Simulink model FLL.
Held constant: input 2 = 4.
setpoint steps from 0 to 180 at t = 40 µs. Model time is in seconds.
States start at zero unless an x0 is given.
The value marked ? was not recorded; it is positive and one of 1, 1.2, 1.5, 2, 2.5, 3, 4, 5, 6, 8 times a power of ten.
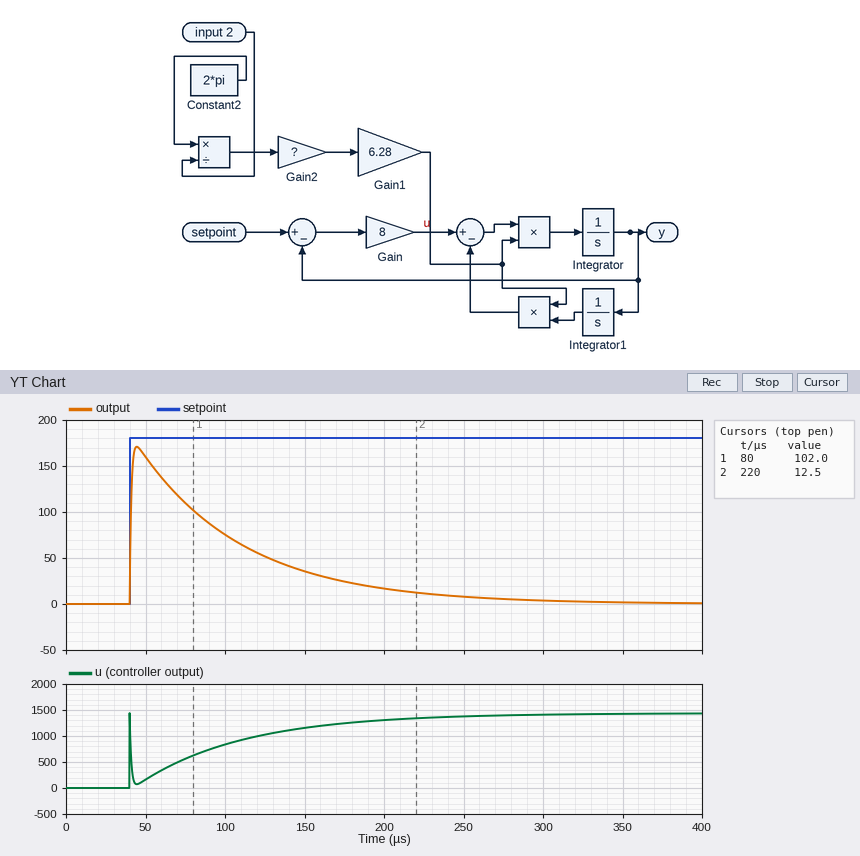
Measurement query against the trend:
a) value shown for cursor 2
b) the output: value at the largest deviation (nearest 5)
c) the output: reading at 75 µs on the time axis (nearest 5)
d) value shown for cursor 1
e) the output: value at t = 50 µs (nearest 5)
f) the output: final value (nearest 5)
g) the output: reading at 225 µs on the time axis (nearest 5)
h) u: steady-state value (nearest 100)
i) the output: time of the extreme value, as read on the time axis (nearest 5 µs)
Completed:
12.5
170
110
102.0
160
0
10
1400
45 µs
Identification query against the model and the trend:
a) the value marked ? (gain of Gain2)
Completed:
12000
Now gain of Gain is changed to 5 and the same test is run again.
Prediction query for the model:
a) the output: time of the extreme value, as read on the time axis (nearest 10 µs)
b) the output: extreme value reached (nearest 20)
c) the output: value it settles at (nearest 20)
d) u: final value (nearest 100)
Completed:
50 µs
160
0
900
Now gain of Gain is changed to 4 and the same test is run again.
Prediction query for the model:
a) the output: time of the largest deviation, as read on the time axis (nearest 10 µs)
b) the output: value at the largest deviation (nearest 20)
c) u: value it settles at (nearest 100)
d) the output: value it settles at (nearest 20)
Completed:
50 µs
160
700
0
